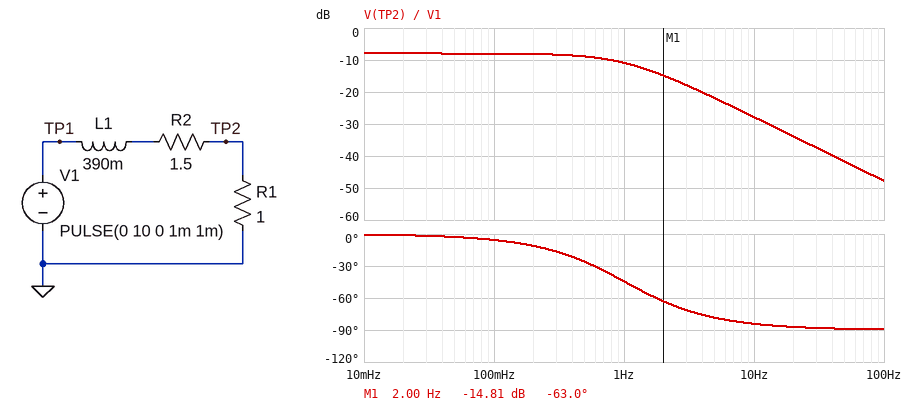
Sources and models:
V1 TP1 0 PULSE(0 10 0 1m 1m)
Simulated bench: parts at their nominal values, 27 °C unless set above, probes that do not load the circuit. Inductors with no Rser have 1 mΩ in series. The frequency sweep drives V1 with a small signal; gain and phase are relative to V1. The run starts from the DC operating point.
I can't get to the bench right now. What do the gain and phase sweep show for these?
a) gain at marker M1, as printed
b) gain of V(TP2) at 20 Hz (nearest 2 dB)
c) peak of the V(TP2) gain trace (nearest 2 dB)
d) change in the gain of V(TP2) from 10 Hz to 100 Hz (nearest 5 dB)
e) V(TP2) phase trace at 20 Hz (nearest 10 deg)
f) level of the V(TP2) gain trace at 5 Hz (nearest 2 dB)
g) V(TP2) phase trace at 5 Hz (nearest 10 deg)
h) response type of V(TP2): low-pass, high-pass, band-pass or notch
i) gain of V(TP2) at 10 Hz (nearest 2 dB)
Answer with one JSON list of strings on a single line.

["-14.81 dB", "-34 dB", "-8 dB", "-20 dB", "-90 deg", "-22 dB", "-80 deg", "low-pass", "-28 dB"]
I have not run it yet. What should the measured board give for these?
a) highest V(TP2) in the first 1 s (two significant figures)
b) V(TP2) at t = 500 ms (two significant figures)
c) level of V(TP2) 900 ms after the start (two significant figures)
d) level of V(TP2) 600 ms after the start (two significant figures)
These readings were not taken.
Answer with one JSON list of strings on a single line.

["4.0 V", "3.8 V", "4.0 V", "3.9 V"]
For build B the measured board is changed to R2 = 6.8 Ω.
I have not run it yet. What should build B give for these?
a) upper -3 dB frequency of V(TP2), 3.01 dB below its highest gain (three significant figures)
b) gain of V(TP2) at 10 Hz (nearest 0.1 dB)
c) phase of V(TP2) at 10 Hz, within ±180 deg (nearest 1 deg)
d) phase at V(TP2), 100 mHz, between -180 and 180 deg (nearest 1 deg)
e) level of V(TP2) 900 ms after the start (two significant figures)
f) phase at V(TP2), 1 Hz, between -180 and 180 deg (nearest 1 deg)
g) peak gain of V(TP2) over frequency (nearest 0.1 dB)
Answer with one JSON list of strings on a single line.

["3.18 Hz", "-28.2 dB", "-72 deg", "-2 deg", "1.3 V", "-17 deg", "-17.8 dB"]
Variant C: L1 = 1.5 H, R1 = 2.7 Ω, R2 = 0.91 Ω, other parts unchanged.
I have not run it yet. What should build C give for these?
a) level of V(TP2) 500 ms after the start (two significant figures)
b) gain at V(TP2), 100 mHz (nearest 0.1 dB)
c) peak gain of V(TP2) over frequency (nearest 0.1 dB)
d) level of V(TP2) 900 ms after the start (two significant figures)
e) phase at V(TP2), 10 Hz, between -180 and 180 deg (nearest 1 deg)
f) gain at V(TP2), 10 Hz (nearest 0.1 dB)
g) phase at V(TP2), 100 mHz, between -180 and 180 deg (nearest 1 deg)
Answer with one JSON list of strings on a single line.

["5.2 V", "-2.8 dB", "-2.5 dB", "6.6 V", "-88 deg", "-30.9 dB", "-15 deg"]
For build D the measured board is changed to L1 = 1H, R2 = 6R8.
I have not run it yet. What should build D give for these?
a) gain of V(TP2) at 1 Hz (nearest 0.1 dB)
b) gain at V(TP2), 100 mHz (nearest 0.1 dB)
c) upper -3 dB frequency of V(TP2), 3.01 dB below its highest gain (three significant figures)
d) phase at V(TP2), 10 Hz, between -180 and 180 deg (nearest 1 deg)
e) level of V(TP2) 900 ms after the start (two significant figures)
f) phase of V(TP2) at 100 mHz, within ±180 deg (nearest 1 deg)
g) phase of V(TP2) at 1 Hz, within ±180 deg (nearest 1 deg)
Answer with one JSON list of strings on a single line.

["-20.0 dB", "-17.9 dB", "1.24 Hz", "-83 deg", "1.3 V", "-5 deg", "-39 deg"]
